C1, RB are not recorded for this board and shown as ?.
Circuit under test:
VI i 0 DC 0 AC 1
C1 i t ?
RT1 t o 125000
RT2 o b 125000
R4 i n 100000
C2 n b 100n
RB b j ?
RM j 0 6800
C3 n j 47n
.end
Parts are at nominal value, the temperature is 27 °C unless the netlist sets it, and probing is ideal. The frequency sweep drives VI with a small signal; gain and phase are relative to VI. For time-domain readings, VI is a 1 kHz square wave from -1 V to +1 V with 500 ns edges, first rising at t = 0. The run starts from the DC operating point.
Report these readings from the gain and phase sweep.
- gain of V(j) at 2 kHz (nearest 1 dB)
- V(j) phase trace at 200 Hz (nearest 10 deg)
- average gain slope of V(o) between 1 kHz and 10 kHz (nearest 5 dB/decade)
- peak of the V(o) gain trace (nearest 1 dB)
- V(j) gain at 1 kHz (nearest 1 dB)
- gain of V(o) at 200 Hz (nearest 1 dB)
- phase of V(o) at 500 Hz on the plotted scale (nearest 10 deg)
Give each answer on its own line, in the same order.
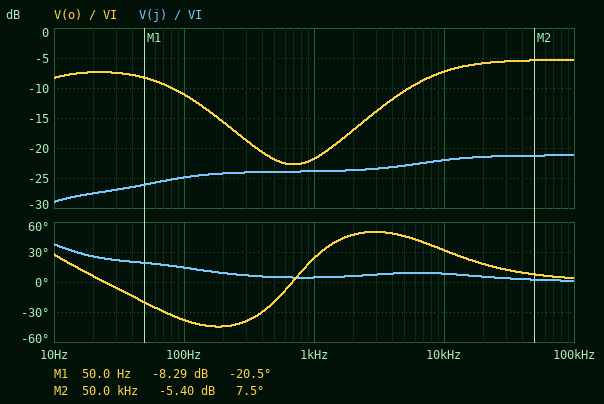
-24 dB
10 deg
15 dB/decade
-5 dB
-24 dB
-16 dB
-20 deg
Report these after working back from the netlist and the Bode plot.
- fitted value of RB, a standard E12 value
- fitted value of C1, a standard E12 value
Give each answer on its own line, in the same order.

100 kΩ
82 pF
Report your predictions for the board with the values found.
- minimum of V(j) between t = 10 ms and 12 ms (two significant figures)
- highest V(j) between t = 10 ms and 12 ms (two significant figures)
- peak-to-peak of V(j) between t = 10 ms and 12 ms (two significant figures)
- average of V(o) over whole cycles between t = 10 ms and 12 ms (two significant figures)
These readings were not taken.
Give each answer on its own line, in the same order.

-88 mV
140 mV
230 mV
310 mV
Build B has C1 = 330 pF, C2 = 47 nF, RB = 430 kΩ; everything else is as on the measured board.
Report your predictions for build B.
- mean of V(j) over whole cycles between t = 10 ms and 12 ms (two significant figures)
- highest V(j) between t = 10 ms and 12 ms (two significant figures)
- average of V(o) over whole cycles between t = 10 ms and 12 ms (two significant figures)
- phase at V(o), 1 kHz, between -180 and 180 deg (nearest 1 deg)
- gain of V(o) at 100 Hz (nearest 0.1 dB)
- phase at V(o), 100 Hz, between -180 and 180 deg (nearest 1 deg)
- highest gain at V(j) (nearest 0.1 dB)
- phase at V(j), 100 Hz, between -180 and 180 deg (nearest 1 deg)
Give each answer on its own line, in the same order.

14 mV
130 mV
550 mV
44 deg
-10.8 dB
-49 deg
-21.2 dB
18 deg
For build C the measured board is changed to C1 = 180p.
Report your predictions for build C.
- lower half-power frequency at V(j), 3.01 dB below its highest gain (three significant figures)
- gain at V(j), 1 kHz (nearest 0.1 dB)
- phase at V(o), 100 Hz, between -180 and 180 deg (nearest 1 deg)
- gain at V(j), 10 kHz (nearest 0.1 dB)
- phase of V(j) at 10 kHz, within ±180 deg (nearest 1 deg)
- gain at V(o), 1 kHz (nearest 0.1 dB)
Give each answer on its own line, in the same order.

206 Hz
-23.7 dB
-37 deg
-21.4 dB
5 deg
-16.9 dB
